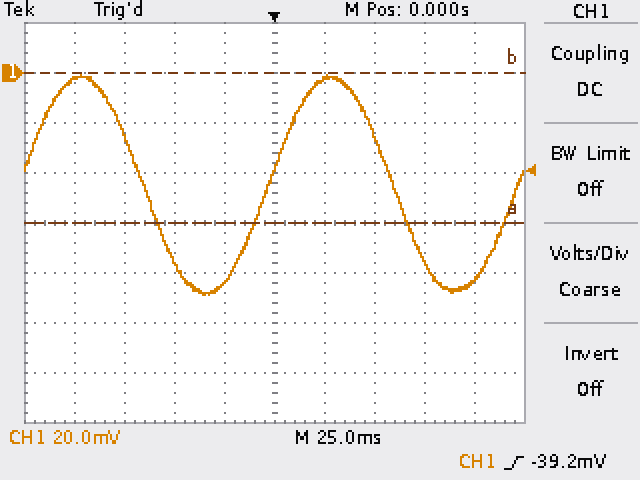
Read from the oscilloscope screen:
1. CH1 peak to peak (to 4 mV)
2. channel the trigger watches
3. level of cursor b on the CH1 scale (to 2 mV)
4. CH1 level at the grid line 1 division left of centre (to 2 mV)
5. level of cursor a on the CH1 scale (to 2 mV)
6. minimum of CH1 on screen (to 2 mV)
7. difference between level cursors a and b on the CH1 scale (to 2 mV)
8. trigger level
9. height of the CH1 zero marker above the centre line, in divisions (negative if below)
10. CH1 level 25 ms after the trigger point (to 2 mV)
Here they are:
88 mV
CH1
0 mV
-84 mV
-60 mV
-88 mV
60 mV
-39.2 mV
+3.0 div
-2 mV
